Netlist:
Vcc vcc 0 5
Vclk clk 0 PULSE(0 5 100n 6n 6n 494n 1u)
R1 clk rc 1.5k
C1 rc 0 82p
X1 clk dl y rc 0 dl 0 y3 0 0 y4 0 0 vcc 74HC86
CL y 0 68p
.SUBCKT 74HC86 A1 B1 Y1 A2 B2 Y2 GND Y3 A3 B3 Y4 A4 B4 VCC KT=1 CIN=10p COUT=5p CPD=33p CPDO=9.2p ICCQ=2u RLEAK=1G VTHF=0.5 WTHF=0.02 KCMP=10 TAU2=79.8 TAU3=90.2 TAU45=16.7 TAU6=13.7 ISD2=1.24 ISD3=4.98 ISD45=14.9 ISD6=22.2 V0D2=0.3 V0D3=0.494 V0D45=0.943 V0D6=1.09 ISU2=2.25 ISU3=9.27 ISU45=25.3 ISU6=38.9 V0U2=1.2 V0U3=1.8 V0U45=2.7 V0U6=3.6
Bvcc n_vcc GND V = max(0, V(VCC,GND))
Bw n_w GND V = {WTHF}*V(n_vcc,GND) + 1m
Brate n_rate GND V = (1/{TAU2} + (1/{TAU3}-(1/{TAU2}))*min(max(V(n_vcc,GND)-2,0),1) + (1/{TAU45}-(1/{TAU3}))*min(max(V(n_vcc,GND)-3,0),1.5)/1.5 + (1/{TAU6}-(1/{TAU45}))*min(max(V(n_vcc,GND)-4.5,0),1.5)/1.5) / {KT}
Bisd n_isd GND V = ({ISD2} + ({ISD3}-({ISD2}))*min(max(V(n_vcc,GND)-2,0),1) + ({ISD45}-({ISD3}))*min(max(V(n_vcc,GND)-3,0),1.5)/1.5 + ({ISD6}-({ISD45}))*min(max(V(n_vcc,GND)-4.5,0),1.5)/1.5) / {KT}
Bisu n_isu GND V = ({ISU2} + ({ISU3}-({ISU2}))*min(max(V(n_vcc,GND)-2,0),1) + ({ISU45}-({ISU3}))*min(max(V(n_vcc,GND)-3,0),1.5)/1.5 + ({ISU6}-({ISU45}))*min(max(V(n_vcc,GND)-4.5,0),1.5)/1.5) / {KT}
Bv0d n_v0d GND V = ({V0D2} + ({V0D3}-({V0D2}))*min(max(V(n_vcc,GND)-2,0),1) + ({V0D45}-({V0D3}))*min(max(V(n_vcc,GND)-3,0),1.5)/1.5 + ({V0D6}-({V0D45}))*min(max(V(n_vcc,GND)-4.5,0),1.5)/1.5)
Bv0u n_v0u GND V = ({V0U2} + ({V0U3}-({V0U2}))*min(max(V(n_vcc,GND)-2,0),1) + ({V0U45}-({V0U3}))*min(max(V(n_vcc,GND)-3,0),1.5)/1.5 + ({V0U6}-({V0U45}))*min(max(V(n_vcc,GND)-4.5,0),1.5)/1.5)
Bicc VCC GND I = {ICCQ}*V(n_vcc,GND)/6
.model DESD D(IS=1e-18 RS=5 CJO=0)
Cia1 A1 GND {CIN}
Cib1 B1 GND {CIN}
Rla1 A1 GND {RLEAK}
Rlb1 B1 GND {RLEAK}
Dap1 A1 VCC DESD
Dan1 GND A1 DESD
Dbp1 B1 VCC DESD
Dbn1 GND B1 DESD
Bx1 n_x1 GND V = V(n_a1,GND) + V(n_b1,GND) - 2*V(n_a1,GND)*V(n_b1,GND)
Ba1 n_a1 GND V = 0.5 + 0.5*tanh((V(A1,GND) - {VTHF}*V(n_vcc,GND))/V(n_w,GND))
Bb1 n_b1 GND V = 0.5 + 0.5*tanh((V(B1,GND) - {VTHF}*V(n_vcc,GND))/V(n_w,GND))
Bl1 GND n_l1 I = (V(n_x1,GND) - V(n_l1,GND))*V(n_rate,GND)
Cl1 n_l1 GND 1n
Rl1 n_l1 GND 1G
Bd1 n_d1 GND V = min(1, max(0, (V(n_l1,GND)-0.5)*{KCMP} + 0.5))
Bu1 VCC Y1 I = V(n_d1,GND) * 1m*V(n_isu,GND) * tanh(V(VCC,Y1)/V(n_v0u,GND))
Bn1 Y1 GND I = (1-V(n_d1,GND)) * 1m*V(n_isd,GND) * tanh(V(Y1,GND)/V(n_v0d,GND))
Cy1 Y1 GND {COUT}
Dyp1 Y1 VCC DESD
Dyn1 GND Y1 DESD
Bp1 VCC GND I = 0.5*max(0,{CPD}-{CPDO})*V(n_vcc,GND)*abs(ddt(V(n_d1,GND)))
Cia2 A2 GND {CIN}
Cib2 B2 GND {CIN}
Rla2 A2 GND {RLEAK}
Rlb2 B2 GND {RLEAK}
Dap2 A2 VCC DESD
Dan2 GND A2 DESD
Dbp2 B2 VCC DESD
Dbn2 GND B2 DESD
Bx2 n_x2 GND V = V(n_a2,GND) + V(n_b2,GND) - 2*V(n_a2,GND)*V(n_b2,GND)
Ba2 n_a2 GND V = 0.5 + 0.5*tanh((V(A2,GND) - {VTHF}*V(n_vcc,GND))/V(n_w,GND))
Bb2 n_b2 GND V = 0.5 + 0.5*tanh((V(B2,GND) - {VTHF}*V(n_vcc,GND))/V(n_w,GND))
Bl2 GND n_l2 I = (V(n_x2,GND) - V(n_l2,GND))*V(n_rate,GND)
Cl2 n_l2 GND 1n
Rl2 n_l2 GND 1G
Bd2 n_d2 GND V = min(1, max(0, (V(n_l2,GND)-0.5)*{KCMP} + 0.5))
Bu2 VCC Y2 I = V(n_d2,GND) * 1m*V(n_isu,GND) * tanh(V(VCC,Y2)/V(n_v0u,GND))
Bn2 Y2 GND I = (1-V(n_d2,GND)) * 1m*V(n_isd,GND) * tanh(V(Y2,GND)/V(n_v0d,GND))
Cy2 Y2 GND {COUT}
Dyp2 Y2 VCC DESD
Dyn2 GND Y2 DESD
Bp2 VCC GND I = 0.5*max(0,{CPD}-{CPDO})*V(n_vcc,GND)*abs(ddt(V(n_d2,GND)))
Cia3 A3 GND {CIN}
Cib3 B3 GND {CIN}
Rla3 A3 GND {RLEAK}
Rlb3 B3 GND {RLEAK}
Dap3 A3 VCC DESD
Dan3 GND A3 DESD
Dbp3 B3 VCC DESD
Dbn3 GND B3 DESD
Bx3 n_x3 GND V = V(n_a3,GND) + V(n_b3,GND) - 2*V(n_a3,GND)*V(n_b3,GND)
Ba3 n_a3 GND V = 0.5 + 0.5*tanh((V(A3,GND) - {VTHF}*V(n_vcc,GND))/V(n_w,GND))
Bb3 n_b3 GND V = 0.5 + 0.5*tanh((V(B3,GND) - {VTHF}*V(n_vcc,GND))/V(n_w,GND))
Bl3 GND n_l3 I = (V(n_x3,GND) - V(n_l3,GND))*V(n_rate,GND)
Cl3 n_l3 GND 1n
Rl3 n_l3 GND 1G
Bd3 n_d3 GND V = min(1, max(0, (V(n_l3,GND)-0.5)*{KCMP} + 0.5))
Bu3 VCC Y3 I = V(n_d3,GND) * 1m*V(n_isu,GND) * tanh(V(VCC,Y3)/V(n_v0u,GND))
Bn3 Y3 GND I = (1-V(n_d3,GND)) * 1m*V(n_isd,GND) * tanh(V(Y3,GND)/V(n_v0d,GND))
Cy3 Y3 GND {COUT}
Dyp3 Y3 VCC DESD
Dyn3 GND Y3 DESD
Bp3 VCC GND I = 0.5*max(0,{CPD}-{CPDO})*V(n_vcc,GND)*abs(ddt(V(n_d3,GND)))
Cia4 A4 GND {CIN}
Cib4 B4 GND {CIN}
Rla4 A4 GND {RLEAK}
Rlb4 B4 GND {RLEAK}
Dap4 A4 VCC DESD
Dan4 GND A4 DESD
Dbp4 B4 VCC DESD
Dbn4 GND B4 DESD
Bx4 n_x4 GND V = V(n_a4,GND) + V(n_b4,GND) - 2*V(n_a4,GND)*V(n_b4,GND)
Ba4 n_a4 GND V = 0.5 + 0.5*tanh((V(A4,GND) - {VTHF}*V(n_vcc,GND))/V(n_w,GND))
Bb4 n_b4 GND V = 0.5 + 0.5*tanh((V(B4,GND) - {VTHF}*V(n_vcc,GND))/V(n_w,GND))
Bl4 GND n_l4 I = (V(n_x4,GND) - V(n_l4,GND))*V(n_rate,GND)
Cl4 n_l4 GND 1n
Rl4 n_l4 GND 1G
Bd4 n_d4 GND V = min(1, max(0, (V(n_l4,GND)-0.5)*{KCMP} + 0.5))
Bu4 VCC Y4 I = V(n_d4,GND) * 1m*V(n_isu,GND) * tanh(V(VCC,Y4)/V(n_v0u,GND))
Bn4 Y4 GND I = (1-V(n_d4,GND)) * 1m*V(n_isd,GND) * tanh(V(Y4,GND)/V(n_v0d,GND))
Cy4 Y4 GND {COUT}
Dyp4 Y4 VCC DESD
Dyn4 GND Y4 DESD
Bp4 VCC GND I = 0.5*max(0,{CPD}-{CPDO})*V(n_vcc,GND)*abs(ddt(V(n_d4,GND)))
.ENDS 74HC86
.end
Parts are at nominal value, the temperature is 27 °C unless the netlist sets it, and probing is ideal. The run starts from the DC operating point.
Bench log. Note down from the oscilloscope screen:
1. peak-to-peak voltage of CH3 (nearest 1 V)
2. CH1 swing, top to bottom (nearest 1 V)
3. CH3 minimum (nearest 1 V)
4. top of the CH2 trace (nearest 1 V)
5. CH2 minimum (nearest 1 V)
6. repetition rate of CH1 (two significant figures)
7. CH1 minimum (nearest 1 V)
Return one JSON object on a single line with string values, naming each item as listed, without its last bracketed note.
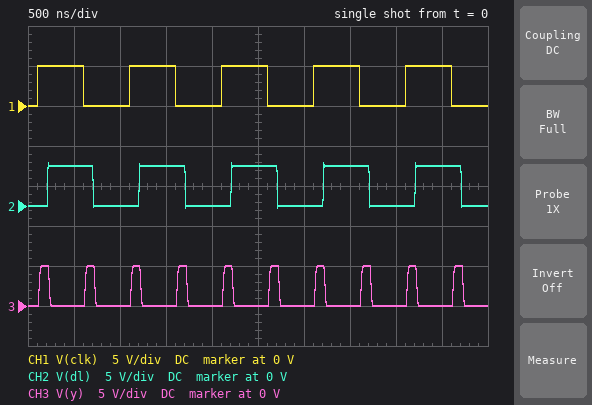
{"peak-to-peak voltage of CH3": "5 V", "CH1 swing, top to bottom": "5 V", "CH3 minimum": "0 V", "top of the CH2 trace": "5 V", "CH2 minimum": "0 V", "repetition rate of CH1": "1.0 MHz", "CH1 minimum": "0 V"}
